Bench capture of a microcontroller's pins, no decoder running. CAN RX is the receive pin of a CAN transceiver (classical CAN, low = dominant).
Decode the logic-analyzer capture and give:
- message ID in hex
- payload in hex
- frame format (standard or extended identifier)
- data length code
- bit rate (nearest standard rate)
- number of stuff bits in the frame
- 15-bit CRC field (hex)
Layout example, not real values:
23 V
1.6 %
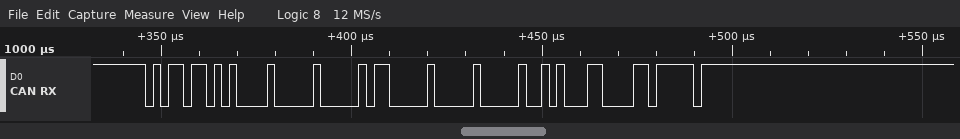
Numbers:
0x5B5
00 60 00 0A
standard
4
500 kbit/s
5
0x186F
